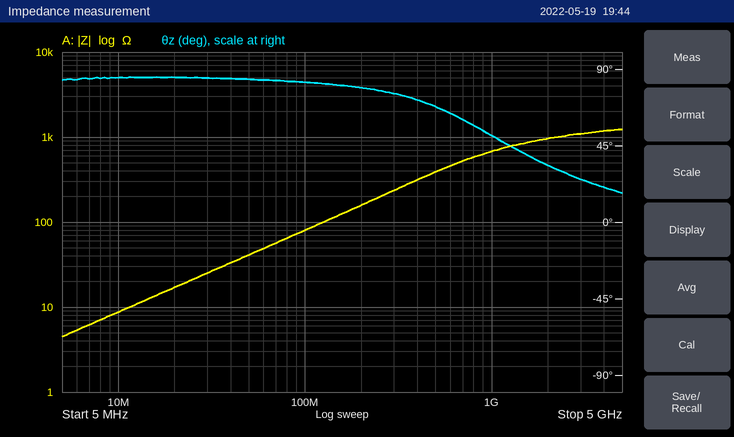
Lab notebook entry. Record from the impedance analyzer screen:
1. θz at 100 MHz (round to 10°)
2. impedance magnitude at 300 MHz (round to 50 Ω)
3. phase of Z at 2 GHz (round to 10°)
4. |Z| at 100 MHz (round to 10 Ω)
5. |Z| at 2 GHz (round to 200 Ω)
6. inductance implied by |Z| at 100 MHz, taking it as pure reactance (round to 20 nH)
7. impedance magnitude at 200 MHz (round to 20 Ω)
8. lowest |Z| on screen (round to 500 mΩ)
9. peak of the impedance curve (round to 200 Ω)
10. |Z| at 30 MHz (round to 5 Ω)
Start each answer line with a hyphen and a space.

- 80°
- 250 Ω
- 30°
- 80 Ω
- 1.0 kΩ
- 120 nH
- 160 Ω
- 4.5 Ω
- 1.2 kΩ
- 25 Ω
